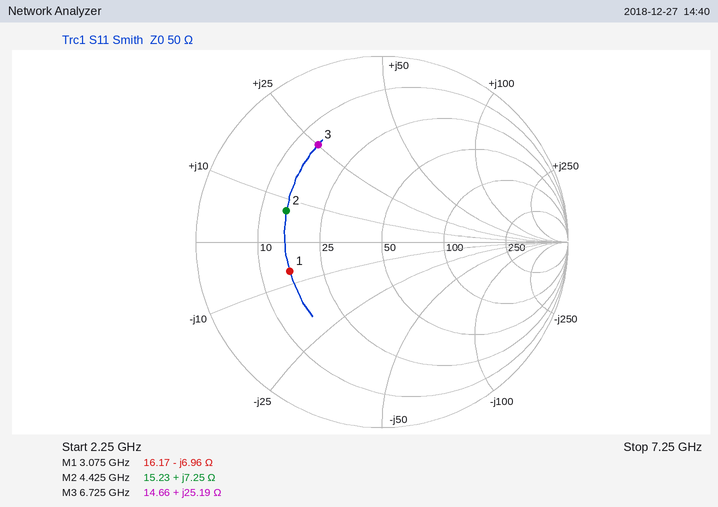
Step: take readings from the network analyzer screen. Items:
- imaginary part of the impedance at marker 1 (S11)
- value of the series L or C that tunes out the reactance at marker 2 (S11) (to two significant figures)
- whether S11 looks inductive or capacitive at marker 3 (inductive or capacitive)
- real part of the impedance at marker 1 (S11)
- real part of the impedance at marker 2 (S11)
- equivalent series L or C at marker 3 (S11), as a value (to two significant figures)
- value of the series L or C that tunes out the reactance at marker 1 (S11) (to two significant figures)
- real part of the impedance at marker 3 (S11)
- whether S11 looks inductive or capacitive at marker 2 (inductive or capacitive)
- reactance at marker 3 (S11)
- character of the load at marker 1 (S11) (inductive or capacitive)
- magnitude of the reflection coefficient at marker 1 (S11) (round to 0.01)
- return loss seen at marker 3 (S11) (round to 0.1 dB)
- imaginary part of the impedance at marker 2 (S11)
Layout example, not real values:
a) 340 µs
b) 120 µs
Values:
a) -6.96 Ω
b) 5.0 pF
c) inductive
d) 16.17 Ω
e) 15.23 Ω
f) 600 pH
g) 360 pH
h) 14.66 Ω
i) inductive
j) +25.19 Ω
k) capacitive
l) 0.52
m) 4.1 dB
n) +7.25 Ω
